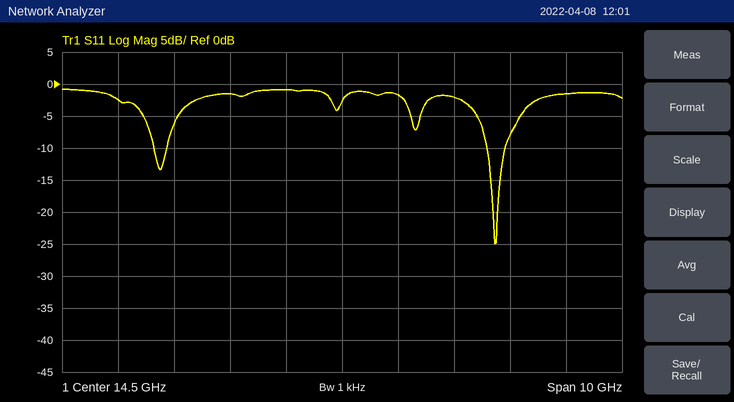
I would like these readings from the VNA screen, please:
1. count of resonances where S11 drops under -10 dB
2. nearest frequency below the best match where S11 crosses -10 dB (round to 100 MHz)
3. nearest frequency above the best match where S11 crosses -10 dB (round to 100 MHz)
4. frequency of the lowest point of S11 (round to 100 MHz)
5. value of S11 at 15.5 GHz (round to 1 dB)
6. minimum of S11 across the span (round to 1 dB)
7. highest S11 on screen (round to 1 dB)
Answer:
2
17.1 GHz
17.4 GHz
17.2 GHz
-2 dB
-25 dB
-1 dB
